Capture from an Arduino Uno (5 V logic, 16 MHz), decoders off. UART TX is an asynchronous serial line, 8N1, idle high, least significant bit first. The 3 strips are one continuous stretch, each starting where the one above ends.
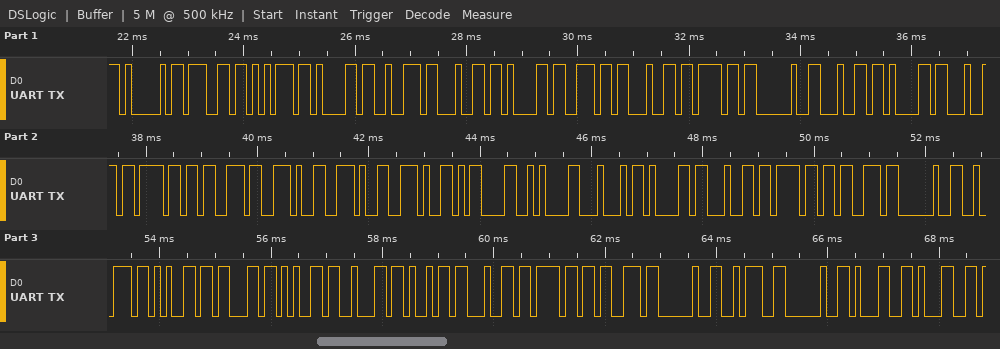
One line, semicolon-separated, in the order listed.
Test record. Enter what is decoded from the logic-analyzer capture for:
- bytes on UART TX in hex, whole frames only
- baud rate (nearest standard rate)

41 67 75 61 72 64 61 6E 64 6F 20 64 61 64 6F 73 2E 2E 2E 0D 0A 44 61 64 6F 73 20 72 65 63 65 62 69 64 6F 73 20 3A 20 31 31; 9600 baud
